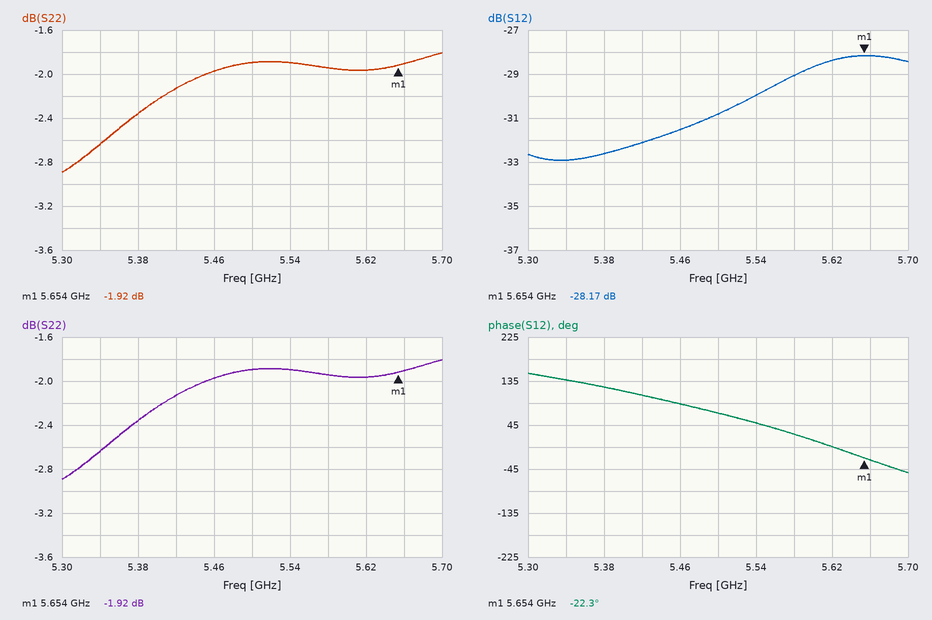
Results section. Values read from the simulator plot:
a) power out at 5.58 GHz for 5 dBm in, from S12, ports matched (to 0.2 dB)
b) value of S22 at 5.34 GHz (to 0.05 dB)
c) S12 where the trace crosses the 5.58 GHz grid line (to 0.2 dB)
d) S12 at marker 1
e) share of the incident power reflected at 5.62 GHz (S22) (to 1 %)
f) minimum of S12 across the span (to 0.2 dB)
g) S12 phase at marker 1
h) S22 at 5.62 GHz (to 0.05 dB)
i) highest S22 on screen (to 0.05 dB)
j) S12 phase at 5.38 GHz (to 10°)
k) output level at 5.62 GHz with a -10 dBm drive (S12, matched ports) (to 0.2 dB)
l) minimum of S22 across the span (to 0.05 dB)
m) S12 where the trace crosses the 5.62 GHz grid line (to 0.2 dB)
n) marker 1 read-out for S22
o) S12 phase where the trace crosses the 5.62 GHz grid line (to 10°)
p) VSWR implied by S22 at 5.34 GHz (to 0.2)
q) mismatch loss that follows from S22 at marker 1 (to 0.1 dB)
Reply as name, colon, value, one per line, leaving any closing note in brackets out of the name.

power out at 5.58 GHz for 5 dBm in, from S12, ports matched: -24.0 dBm
value of S22 at 5.34 GHz: -2.65 dB
S12 where the trace crosses the 5.58 GHz grid line: -29.0 dB
S12 at marker 1: -28.17 dB
share of the incident power reflected at 5.62 GHz (S22): 64 %
minimum of S12 across the span: -33.0 dB
S12 phase at marker 1: -22.3°
S22 at 5.62 GHz: -1.95 dB
highest S22 on screen: -1.80 dB
S12 phase at 5.38 GHz: 120°
output level at 5.62 GHz with a -10 dBm drive (S12, matched ports): -38.4 dBm
minimum of S22 across the span: -2.90 dB
S12 where the trace crosses the 5.62 GHz grid line: -28.4 dB
marker 1 read-out for S22: -1.92 dB
S12 phase where the trace crosses the 5.62 GHz grid line: 0°
VSWR implied by S22 at 5.34 GHz: 6.6
mismatch loss that follows from S22 at marker 1: 4.5 dB
